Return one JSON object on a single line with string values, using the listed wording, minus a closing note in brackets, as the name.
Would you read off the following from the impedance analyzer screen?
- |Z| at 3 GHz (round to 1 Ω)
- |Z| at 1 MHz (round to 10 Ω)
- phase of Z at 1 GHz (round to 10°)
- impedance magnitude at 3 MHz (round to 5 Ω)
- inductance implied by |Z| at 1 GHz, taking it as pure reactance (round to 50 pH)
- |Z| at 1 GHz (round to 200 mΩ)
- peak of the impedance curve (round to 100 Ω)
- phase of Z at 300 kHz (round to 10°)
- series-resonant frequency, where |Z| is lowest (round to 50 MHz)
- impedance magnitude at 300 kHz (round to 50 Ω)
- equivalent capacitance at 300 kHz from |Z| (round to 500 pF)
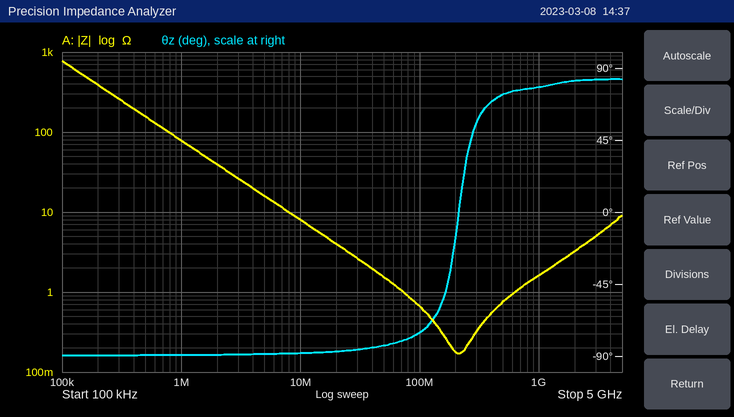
{"|Z| at 3 GHz": "5 Ω", "|Z| at 1 MHz": "80 Ω", "phase of Z at 1 GHz": "80°", "impedance magnitude at 3 MHz": "25 Ω", "inductance implied by |Z| at 1 GHz, taking it as pure reactance": "250 pH", "|Z| at 1 GHz": "1.6 Ω", "peak of the impedance curve": "800 Ω", "phase of Z at 300 kHz": "-90°", "series-resonant frequency, where |Z| is lowest": "200 MHz", "impedance magnitude at 300 kHz": "250 Ω", "equivalent capacitance at 300 kHz from |Z|": "2.0 nF"}
